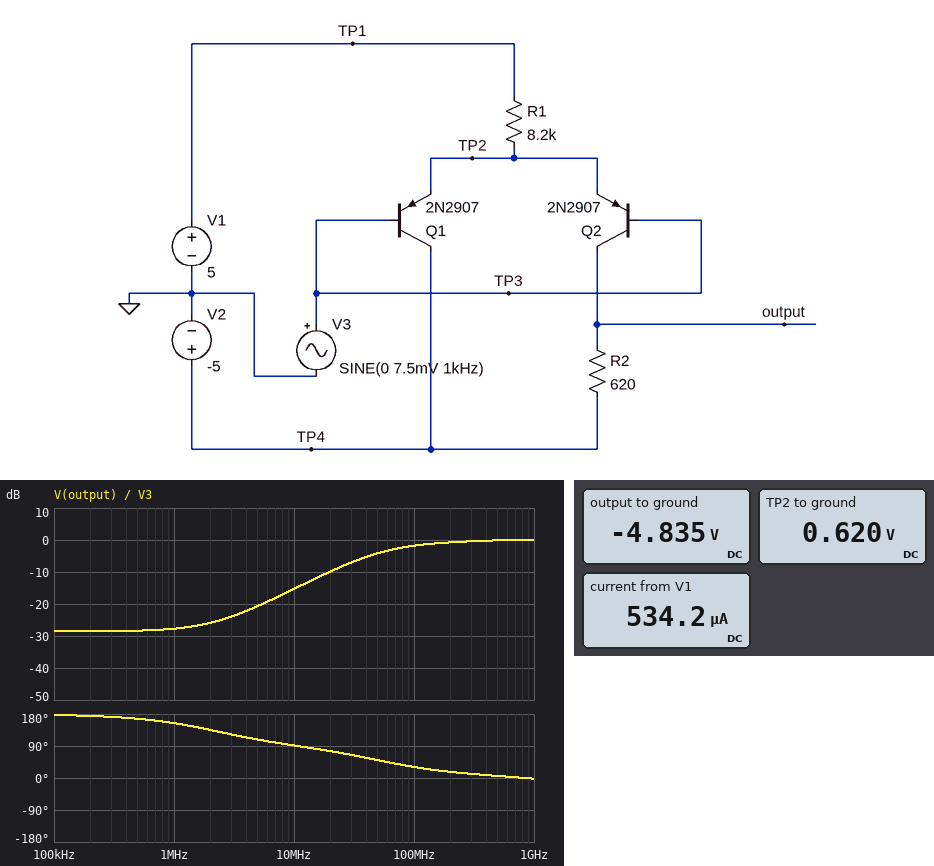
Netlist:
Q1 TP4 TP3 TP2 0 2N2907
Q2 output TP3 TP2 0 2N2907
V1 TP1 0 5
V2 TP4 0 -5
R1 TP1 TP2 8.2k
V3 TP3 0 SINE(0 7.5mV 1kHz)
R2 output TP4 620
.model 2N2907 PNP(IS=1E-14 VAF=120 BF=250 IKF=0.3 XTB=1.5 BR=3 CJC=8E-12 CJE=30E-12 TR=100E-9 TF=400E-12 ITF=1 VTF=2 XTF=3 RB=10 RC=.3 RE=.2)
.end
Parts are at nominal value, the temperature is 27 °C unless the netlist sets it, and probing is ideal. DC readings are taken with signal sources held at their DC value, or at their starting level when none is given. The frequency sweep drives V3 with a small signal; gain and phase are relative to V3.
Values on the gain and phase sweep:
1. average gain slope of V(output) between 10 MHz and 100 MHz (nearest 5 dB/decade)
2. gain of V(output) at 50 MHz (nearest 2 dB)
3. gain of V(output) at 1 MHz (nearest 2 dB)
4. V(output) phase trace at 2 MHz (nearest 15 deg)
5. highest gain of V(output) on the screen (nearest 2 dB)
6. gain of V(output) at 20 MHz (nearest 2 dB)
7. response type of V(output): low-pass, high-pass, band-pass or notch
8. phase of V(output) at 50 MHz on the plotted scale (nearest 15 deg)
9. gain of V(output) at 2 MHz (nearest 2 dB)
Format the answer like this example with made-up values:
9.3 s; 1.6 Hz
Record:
15 dB/decade; -4 dB; -28 dB; 135 deg; 0 dB; -10 dB; high-pass; 45 deg; -26 dB
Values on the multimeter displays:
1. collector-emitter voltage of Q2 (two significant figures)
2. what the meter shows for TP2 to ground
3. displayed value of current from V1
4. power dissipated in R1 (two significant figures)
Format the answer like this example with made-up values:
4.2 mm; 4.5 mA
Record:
-5.5 V; 0.620 V; 534.2 µA; 2.3 mW
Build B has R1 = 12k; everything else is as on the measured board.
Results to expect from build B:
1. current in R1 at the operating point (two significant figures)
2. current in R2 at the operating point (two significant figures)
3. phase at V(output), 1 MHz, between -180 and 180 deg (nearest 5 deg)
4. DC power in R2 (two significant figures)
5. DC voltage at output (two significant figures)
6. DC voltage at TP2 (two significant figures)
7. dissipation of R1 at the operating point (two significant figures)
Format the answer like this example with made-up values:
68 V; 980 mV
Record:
370 µA; 180 µA; 145 deg; 21 µW; -4.9 V; 610 mV; 1.6 mW
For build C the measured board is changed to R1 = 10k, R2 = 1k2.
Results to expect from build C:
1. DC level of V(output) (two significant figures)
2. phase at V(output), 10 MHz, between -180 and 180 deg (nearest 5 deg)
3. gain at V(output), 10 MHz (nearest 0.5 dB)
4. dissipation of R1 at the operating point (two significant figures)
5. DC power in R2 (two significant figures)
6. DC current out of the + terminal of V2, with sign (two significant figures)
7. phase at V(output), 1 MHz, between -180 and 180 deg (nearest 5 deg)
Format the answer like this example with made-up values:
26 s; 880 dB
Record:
-4.7 V; 80 deg; -10.0 dB; 1.9 mW; 57 µW; -440 µA; 150 deg
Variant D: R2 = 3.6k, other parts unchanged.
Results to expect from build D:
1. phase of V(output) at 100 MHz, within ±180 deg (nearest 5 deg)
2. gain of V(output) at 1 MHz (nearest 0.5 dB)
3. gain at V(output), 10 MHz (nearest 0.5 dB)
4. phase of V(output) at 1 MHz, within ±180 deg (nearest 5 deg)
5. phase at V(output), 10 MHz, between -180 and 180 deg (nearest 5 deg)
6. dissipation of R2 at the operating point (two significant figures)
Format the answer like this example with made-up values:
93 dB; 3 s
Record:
5 deg; -12.5 dB; -2.5 dB; 150 deg; 55 deg; 250 µW
